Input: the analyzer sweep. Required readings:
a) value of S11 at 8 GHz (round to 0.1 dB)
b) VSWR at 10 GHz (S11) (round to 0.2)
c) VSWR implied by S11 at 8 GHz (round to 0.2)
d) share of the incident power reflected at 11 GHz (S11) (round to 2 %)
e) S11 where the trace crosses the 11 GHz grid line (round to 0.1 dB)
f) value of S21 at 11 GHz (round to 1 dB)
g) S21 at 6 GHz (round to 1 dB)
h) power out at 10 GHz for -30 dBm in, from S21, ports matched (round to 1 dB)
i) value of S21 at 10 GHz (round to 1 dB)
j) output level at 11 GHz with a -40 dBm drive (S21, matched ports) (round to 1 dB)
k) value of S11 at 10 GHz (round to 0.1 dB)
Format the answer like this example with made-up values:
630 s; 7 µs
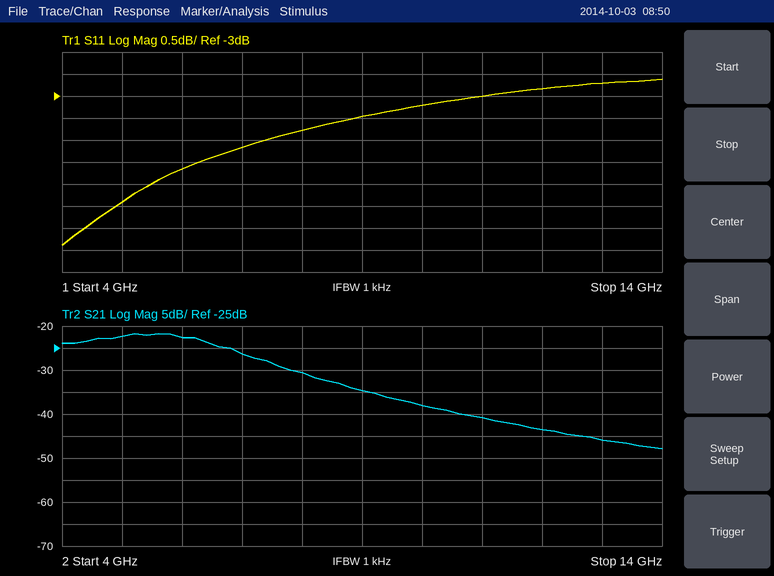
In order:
-3.8 dB; 5.4; 4.6; 50 %; -3.0 dB; -41 dB; -23 dB; -68 dBm; -38 dB; -81 dBm; -3.2 dB
